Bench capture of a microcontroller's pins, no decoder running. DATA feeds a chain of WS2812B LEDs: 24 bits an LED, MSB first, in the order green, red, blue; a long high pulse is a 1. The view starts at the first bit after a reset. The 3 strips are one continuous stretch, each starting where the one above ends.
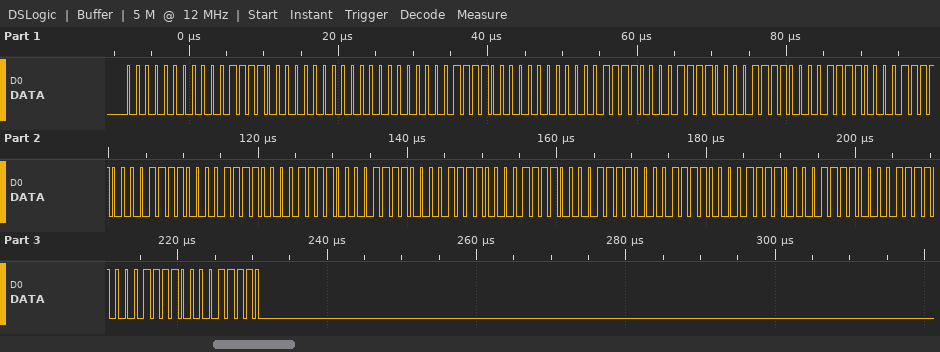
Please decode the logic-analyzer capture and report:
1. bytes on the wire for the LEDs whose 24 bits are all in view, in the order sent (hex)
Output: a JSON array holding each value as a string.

["00 1E 00 00 1E 00 1E 1E 1E 1E 1E 1E 1E 1E 1E 1E 1E 1E 1E 1E 1E 1E 1E 1E"]
